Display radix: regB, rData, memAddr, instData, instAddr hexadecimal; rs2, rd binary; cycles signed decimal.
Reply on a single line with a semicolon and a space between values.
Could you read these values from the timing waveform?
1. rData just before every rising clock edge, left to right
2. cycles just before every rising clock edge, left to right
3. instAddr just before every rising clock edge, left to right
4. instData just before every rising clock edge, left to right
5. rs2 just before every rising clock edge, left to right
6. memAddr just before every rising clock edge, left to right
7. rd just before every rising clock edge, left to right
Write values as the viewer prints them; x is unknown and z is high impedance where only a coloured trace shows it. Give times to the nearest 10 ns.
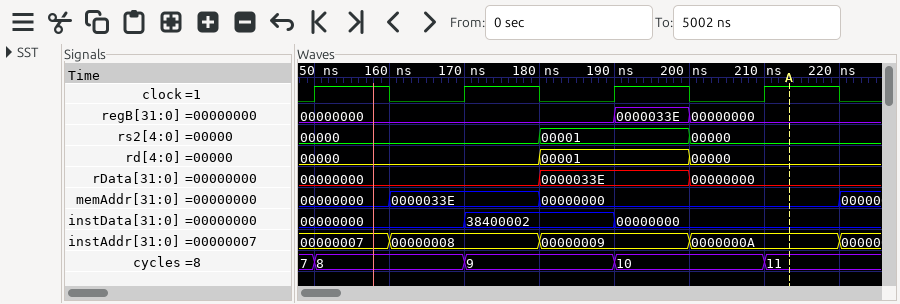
00000000, 00000000, 0000033E, 00000000; 7, 8, 9, 10; 00000007, 00000008, 00000009, 0000000A; 00000000, 00000000, 38400002, 00000000; 00000, 00000, 00001, 00000; 00000000, 0000033E, 00000000, 00000000; 00000, 00000, 00001, 00000
